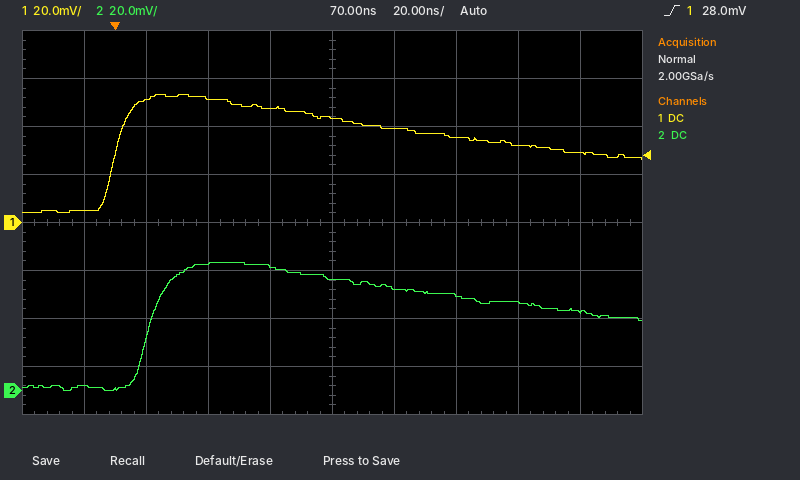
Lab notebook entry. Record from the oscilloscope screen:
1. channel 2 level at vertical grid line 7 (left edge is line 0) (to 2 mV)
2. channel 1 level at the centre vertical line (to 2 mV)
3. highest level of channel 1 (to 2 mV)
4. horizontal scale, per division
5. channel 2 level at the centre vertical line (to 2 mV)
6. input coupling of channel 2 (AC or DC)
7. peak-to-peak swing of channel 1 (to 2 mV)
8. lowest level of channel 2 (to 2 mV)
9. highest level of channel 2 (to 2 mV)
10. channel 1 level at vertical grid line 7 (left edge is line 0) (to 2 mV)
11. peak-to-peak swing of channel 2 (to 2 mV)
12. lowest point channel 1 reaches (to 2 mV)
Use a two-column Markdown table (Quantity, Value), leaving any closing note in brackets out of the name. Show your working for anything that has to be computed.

| Quantity | Value |
|---|---|
| channel 2 level at vertical grid line 7 (left edge is line 0) | 40 mV |
| channel 1 level at the centre vertical line | 44 mV |
| highest level of channel 1 | 54 mV |
| horizontal scale, per division | 20 ns |
| channel 2 level at the centre vertical line | 46 mV |
| input coupling of channel 2 | DC |
| peak-to-peak swing of channel 1 | 54 mV − (4 mV) = 50 mV |
| lowest level of channel 2 | 0 mV |
| highest level of channel 2 | 54 mV |
| channel 1 level at vertical grid line 7 (left edge is line 0) | 36 mV |
| peak-to-peak swing of channel 2 | 54 mV − (0 mV) = 54 mV |
| lowest point channel 1 reaches | 4 mV |
